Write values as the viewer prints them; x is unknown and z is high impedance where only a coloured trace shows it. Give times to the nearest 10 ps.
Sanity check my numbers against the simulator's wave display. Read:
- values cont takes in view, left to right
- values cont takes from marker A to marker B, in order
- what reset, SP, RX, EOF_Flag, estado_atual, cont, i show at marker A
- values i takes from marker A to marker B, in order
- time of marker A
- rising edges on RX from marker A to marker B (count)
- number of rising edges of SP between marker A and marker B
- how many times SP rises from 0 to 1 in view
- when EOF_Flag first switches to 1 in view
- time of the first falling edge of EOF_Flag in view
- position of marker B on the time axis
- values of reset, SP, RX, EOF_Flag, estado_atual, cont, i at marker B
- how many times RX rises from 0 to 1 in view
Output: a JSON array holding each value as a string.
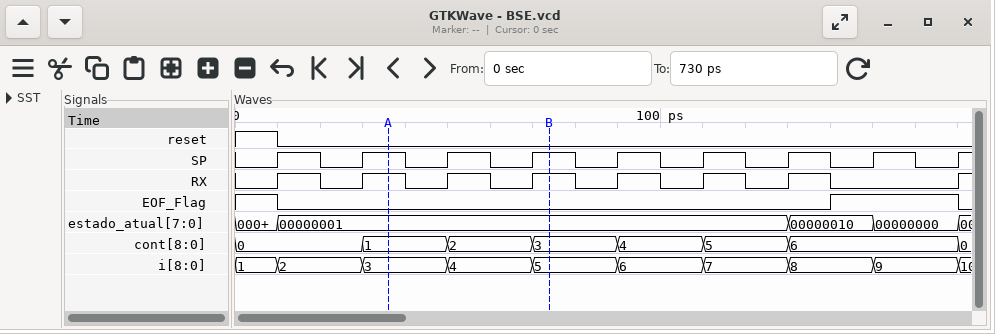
["0, 1, 2, 3, 4, 5, 6, 0", "1, 2, 3", "reset=0, SP=1, RX=1, EOF_Flag=0, estado_atual=00000001, cont=1, i=3", "3, 4, 5", "40 ps", "2", "2", "9", "140 ps", "10 ps", "70 ps", "reset=0, SP=1, RX=1, EOF_Flag=0, estado_atual=00000001, cont=3, i=5", "8"]
